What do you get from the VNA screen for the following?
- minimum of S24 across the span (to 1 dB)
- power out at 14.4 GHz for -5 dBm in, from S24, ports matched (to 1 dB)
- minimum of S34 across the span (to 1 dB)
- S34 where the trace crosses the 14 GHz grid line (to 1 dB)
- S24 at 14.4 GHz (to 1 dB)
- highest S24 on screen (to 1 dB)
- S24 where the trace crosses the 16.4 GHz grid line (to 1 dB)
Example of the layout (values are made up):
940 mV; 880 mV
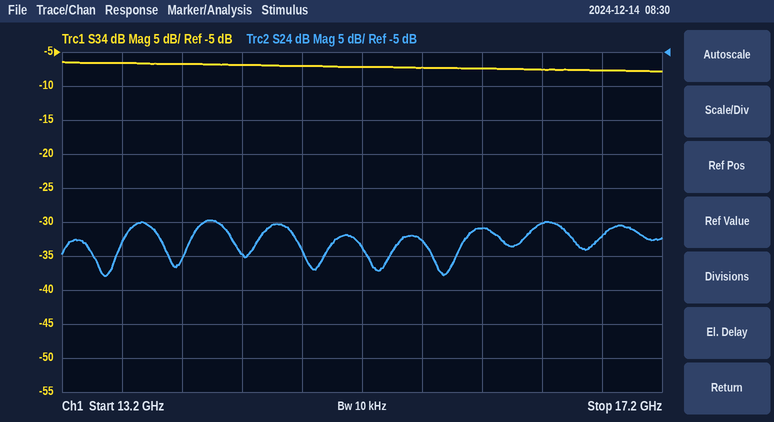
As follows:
-38 dB; -40 dBm; -8 dB; -7 dB; -35 dB; -30 dB; -30 dB
